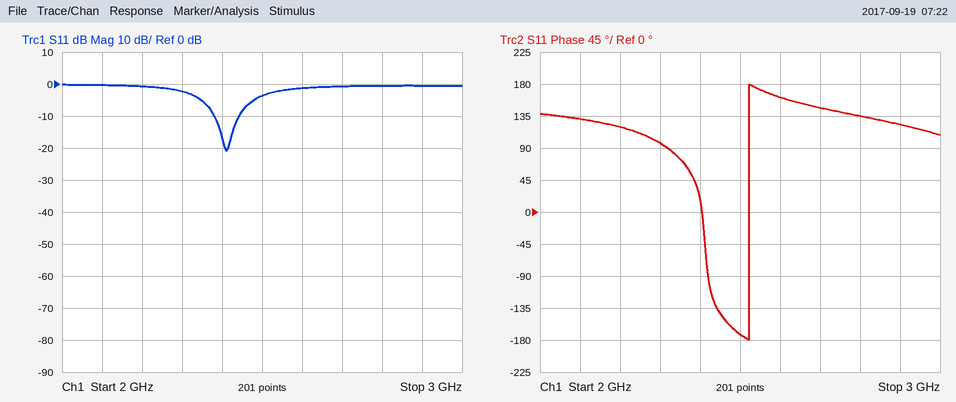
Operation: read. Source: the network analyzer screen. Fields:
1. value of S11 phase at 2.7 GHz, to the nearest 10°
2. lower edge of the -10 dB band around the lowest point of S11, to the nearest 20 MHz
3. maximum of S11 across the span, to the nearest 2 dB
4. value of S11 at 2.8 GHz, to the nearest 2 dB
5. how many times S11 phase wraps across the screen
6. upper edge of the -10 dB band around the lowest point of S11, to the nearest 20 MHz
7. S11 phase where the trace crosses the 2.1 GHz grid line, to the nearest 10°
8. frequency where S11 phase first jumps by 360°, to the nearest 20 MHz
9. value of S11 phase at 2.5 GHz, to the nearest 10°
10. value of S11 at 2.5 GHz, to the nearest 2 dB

150°
2.38 GHz
0 dB
0 dB
1
2.44 GHz
130°
2.52 GHz
-170°
-4 dB
